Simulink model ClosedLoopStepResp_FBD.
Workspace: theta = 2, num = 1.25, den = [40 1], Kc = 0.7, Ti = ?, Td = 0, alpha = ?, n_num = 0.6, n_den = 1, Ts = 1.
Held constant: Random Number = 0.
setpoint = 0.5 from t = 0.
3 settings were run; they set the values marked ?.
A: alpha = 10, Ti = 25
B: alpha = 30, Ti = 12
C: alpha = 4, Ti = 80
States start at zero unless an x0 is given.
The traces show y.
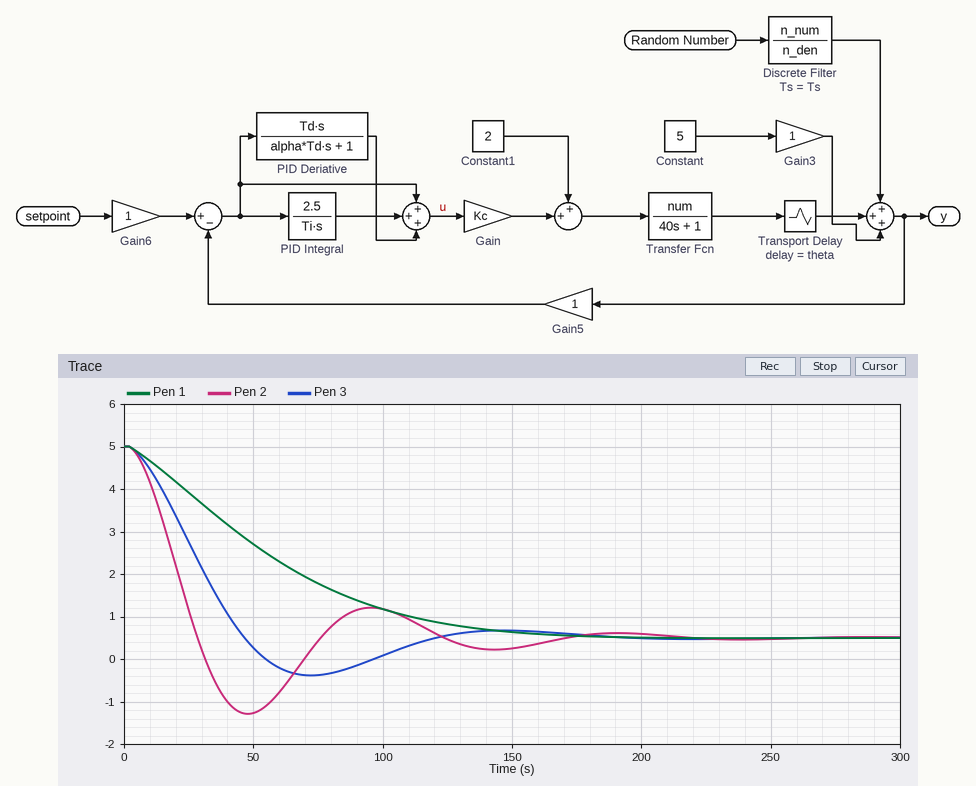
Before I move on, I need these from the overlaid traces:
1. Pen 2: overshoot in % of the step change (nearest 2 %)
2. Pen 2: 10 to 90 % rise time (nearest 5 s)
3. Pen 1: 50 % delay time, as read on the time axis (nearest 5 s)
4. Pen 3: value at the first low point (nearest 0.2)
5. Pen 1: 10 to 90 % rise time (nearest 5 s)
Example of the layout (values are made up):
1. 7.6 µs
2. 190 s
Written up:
1. 40 %
2. 20 s
3. 50 s
4. -0.4
5. 100 s
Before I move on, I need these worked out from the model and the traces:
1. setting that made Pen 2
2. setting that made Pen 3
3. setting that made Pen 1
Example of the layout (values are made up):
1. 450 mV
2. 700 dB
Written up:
1. B
2. A
3. C
